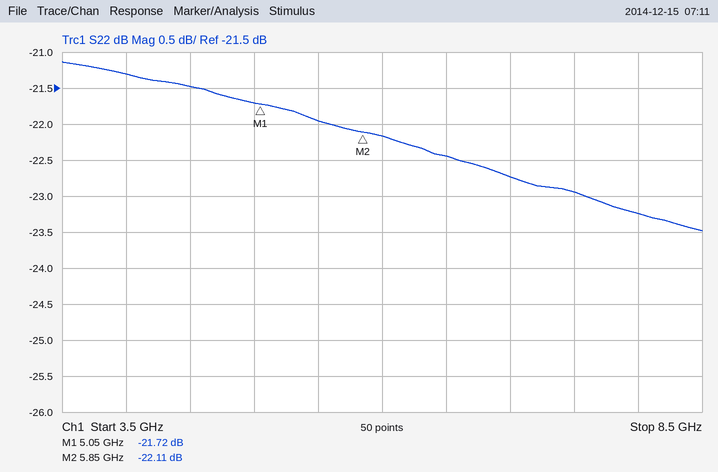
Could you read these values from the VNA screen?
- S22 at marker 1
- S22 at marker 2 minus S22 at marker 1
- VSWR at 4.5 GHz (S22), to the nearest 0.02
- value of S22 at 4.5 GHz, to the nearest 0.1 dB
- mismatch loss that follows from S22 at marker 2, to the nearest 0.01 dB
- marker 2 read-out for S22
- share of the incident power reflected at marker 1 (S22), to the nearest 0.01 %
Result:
-21.72 dB
-0.39 dB
1.18
-21.5 dB
0.03 dB
-22.11 dB
0.67 %
